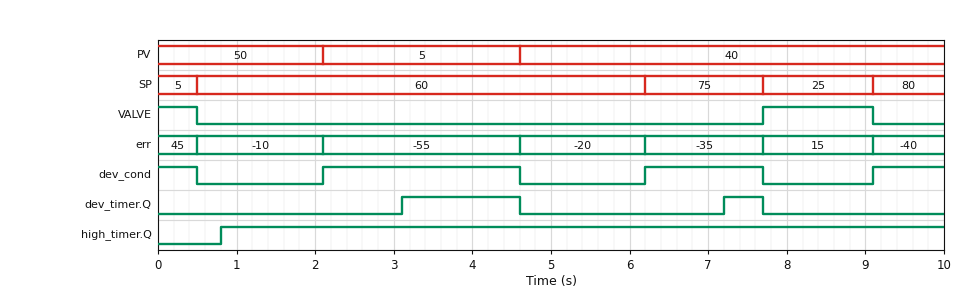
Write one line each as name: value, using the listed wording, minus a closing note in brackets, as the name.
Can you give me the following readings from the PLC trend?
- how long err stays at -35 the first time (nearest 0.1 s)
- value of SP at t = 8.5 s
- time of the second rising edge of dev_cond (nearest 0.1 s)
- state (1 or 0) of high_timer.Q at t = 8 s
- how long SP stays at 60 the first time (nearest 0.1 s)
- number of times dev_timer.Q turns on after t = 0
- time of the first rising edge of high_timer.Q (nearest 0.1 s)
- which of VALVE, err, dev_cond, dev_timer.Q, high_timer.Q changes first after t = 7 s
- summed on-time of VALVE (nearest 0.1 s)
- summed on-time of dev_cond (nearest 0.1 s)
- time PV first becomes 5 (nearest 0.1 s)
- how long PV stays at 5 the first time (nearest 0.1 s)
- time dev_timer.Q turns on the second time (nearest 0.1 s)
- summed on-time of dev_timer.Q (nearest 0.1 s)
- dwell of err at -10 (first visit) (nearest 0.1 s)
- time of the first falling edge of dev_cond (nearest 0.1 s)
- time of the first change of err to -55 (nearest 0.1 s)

how long err stays at -35 the first time: 1.5 s
value of SP at t = 8.5 s: 25
time of the second rising edge of dev_cond: 6.2 s
state (1 or 0) of high_timer.Q at t = 8 s: 1
how long SP stays at 60 the first time: 5.7 s
number of times dev_timer.Q turns on after t = 0: 2
time of the first rising edge of high_timer.Q: 0.8 s
which of VALVE, err, dev_cond, dev_timer.Q, high_timer.Q changes first after t = 7 s: dev_timer.Q
summed on-time of VALVE: 1.9 s
summed on-time of dev_cond: 5.4 s
time PV first becomes 5: 2.1 s
how long PV stays at 5 the first time: 2.5 s
time dev_timer.Q turns on the second time: 7.2 s
summed on-time of dev_timer.Q: 2.0 s
dwell of err at -10 (first visit): 1.6 s
time of the first falling edge of dev_cond: 0.5 s
time of the first change of err to -55: 2.1 s
